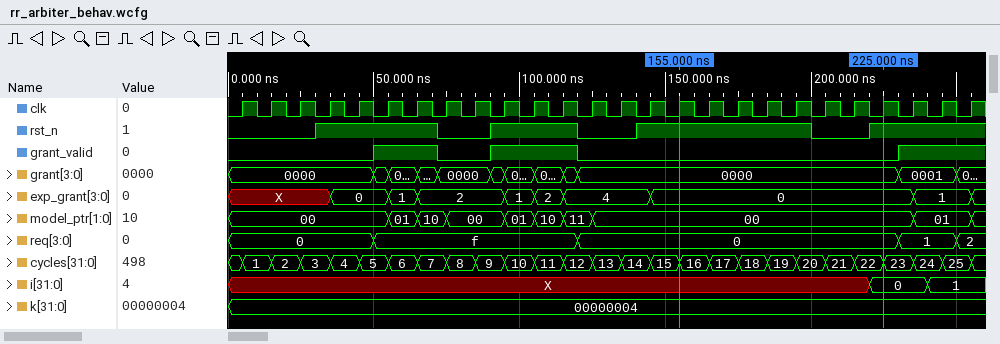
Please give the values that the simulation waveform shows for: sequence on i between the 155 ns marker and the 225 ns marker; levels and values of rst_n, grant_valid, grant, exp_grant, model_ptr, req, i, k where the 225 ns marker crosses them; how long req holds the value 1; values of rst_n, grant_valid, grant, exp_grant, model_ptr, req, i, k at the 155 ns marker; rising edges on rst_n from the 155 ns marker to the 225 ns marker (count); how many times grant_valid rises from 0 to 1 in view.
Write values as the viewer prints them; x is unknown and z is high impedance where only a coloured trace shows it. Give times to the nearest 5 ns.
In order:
X, 0
rst_n=1, grant_valid=0, grant=0000, exp_grant=0, model_ptr=00, req=0, i=0, k=00000004
20 ns
rst_n=1, grant_valid=0, grant=0000, exp_grant=0, model_ptr=00, req=0, i=X, k=00000004
1
3
